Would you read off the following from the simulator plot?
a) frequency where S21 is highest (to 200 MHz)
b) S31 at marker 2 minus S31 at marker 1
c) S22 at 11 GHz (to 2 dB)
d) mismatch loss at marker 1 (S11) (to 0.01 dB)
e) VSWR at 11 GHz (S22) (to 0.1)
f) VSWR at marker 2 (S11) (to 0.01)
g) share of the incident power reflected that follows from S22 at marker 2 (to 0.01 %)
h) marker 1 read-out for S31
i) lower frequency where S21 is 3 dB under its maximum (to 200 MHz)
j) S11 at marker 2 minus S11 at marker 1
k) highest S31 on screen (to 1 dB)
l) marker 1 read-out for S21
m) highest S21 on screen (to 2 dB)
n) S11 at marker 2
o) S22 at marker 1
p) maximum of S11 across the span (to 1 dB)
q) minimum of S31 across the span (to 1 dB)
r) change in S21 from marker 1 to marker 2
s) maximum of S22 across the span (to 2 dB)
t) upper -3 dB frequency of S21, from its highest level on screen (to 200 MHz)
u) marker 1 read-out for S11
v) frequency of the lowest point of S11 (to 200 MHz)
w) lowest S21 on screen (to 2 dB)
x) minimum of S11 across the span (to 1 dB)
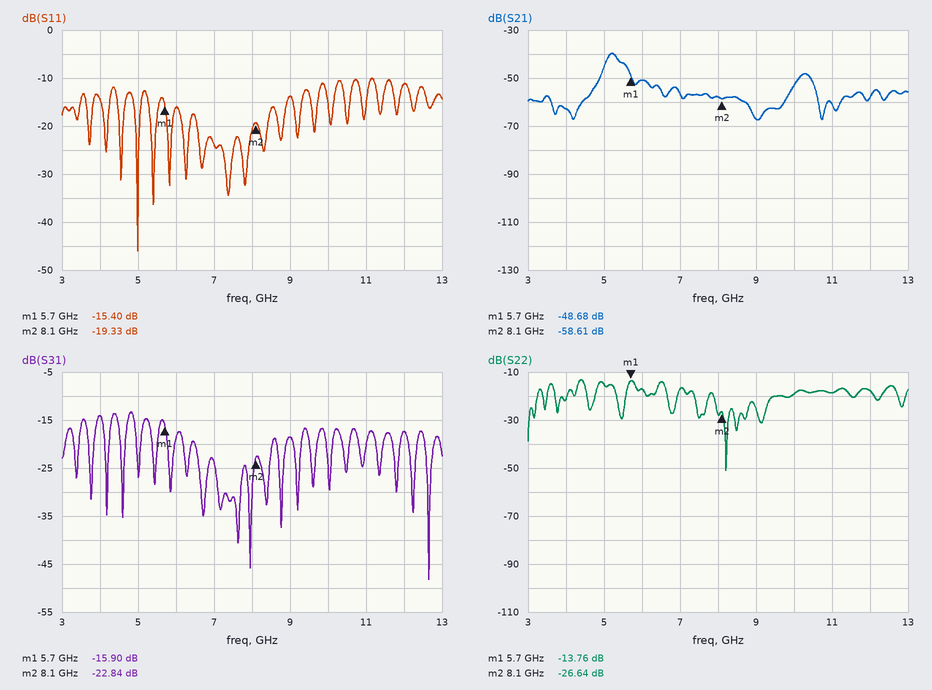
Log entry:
5.2 GHz
-6.94 dB
-18 dB
0.13 dB
1.3
1.24
0.22 %
-15.90 dB
5.0 GHz
-3.93 dB
-13 dB
-48.68 dB
-40 dB
-19.33 dB
-13.76 dB
-10 dB
-48 dB
-9.93 dB
-14 dB
5.4 GHz
-15.40 dB
5.0 GHz
-68 dB
-46 dB
